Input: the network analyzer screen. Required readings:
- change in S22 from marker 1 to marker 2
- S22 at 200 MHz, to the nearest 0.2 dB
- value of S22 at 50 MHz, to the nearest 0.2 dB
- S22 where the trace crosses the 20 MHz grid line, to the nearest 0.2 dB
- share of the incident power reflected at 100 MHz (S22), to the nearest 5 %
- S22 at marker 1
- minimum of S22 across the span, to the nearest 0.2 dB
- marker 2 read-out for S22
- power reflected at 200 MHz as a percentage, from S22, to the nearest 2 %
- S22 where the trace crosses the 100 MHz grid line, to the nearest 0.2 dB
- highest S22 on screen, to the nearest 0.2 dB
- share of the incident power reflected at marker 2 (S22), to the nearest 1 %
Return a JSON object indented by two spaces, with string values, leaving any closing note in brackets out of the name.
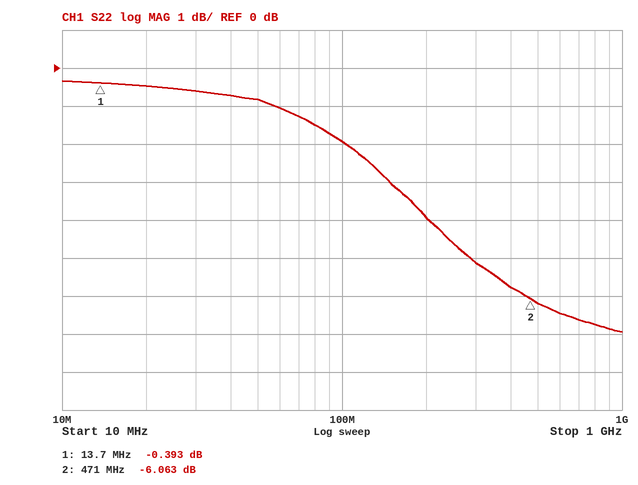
{
  "change in S22 from marker 1 to marker 2": "-5.670 dB",
  "S22 at 200 MHz, to the nearest 0.2 dB": "-4.0 dB",
  "value of S22 at 50 MHz, to the nearest 0.2 dB": "-0.8 dB",
  "S22 where the trace crosses the 20 MHz grid line, to the nearest 0.2 dB": "-0.4 dB",
  "share of the incident power reflected at 100 MHz (S22), to the nearest 5 %": "65 %",
  "S22 at marker 1": "-0.393 dB",
  "minimum of S22 across the span, to the nearest 0.2 dB": "-7.0 dB",
  "marker 2 read-out for S22": "-6.063 dB",
  "power reflected at 200 MHz as a percentage, from S22, to the nearest 2 %": "40 %",
  "S22 where the trace crosses the 100 MHz grid line, to the nearest 0.2 dB": "-2.0 dB",
  "highest S22 on screen, to the nearest 0.2 dB": "-0.4 dB",
  "share of the incident power reflected at marker 2 (S22), to the nearest 1 %": "25 %"
}
